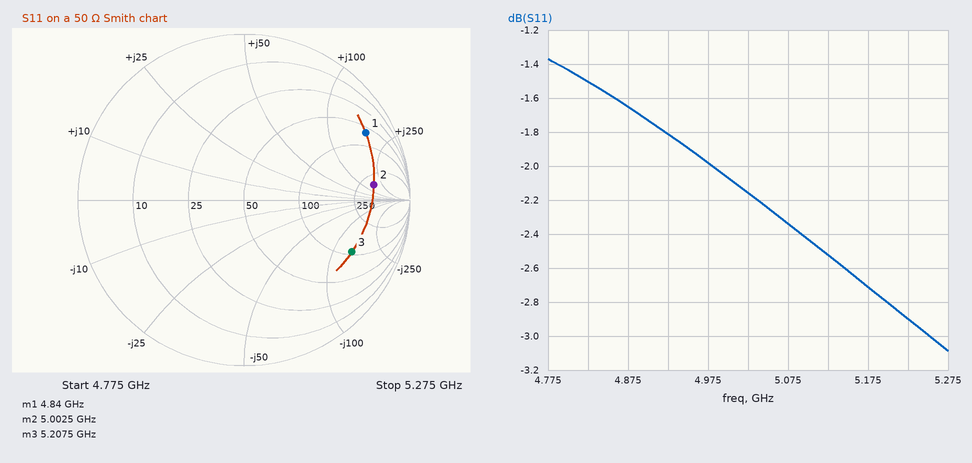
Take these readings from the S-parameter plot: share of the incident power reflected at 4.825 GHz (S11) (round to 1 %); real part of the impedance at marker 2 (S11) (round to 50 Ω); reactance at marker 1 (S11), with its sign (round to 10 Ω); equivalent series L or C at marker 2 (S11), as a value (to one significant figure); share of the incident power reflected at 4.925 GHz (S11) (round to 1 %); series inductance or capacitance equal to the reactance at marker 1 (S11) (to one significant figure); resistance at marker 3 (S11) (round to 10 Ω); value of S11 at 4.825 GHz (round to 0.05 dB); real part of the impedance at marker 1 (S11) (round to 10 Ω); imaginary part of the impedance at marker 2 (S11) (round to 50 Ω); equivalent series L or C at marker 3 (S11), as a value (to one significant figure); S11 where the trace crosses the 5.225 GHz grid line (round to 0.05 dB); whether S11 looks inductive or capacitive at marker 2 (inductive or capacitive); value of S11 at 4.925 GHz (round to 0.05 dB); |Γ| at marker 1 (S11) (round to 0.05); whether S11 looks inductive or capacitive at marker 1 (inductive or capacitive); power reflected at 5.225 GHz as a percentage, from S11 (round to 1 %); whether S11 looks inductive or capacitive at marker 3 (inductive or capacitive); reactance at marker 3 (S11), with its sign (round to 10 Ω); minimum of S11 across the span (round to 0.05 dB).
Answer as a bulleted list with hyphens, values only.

- 71 %
- 350 Ω
- +170 Ω
- 5 nH
- 66 %
- 6 nH
- 110 Ω
- -1.50 dB
- 60 Ω
- +150 Ω
- 200 fF
- -2.90 dB
- inductive
- -1.80 dB
- 0.85
- inductive
- 51 %
- capacitive
- -140 Ω
- -3.10 dB
